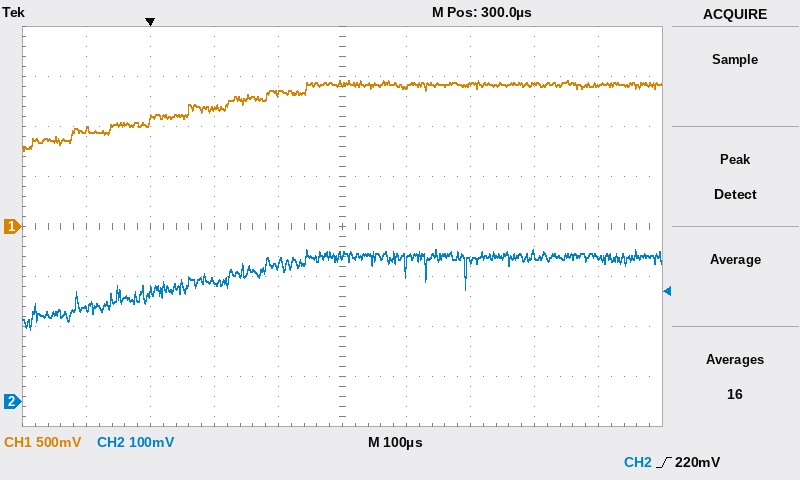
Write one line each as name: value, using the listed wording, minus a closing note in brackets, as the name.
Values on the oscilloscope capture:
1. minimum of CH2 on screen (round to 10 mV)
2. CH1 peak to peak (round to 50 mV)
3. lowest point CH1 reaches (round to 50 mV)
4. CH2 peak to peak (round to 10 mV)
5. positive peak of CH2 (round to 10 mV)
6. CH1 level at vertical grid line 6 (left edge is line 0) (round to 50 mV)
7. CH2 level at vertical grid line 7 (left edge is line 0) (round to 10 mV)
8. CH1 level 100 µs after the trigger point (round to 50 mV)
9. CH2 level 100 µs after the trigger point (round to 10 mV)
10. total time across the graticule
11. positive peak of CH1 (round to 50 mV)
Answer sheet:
minimum of CH2 on screen: 140 mV
CH1 peak to peak: 700 mV
lowest point CH1 reaches: 750 mV
CH2 peak to peak: 160 mV
positive peak of CH2: 300 mV
CH1 level at vertical grid line 6 (left edge is line 0): 1.40 V
CH2 level at vertical grid line 7 (left edge is line 0): 280 mV
CH1 level 100 µs after the trigger point: 1.20 V
CH2 level 100 µs after the trigger point: 240 mV
total time across the graticule: 1 ms
positive peak of CH1: 1.45 V
